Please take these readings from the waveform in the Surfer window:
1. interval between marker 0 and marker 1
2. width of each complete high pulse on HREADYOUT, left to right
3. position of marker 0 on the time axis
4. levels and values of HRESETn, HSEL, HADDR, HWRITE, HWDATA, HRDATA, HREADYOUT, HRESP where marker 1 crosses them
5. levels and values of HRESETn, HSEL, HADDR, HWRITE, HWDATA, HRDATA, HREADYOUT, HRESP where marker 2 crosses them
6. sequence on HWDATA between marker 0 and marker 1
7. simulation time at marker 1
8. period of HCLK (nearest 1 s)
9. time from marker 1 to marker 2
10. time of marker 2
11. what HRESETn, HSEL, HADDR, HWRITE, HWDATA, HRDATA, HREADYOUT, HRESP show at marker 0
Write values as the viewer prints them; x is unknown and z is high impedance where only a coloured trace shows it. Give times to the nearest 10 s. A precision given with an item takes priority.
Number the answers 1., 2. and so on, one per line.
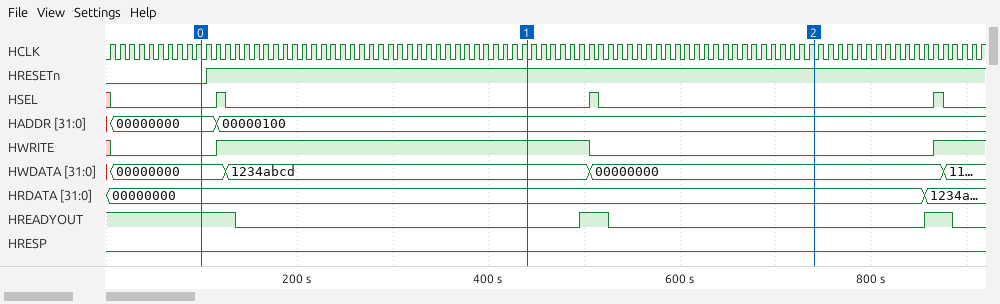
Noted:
1. 340 s
2. 30 s, 30 s
3. 100 s
4. HRESETn=1, HSEL=0, HADDR=00000100, HWRITE=1, HWDATA=1234abcd, HRDATA=00000000, HREADYOUT=0, HRESP=0
5. HRESETn=1, HSEL=0, HADDR=00000100, HWRITE=0, HWDATA=00000000, HRDATA=00000000, HREADYOUT=0, HRESP=0
6. 00000000, 1234abcd
7. 440 s
8. 10 s
9. 300 s
10. 740 s
11. HRESETn=0, HSEL=0, HADDR=00000000, HWRITE=0, HWDATA=00000000, HRDATA=00000000, HREADYOUT=1, HRESP=0
